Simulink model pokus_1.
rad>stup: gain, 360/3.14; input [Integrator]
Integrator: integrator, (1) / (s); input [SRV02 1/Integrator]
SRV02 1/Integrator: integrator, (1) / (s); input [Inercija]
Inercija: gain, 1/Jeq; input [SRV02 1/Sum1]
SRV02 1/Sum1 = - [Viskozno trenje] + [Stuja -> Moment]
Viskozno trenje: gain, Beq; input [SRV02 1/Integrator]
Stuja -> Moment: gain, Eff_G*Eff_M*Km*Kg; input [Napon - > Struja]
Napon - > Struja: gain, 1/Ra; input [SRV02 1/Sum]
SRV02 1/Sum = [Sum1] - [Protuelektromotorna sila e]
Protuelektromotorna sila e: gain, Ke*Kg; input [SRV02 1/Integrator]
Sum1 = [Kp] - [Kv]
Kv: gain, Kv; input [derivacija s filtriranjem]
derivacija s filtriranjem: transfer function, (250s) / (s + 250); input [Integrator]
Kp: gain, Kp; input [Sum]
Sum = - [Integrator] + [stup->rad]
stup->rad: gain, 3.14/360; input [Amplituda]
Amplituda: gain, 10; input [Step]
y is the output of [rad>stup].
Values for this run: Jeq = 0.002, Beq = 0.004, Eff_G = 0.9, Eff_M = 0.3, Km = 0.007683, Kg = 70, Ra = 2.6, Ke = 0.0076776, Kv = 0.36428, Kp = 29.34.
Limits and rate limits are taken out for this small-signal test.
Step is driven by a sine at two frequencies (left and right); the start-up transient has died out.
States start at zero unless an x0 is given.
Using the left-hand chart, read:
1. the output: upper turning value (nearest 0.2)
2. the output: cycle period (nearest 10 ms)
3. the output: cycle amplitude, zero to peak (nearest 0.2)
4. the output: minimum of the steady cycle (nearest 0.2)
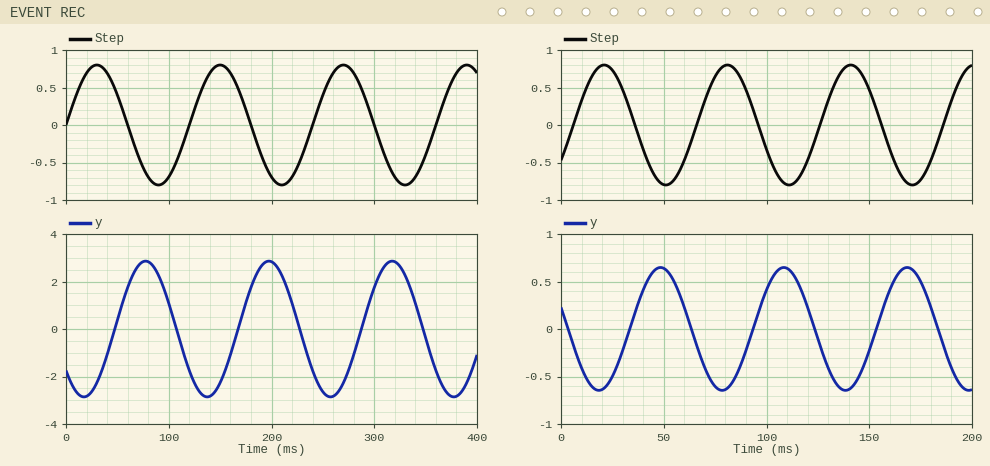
2.8
120 ms
2.8
-2.8
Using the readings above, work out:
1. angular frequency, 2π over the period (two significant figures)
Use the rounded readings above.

0.052 rad/ms
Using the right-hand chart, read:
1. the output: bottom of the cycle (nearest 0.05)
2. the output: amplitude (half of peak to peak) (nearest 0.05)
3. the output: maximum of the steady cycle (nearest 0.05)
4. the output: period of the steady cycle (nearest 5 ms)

-0.65
0.65
0.65
60 ms
